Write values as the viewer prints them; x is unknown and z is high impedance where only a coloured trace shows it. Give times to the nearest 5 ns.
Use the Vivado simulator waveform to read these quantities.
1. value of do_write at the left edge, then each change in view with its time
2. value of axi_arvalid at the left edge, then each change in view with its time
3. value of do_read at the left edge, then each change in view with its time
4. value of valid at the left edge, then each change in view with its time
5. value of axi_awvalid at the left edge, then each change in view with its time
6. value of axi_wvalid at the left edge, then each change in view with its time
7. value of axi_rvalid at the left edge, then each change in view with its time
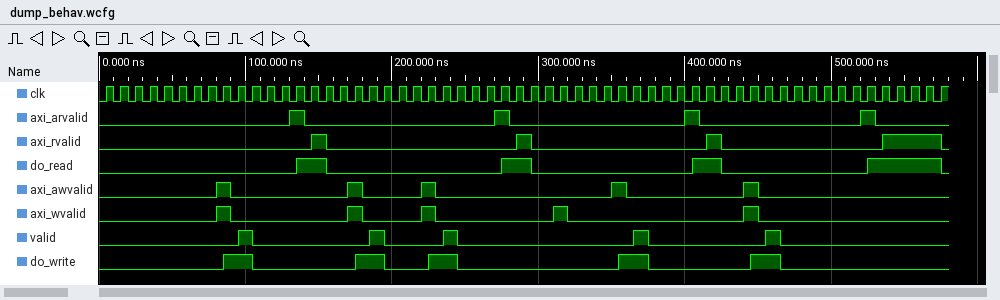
0, 1 at 85 ns, 0 at 105 ns, 1 at 175 ns, 0 at 195 ns, 1 at 225 ns, 0 at 245 ns, 1 at 355 ns, 0 at 375 ns, 1 at 445 ns, 0 at 465 ns
0, 1 at 130 ns, 0 at 140 ns, 1 at 270 ns, 0 at 280 ns, 1 at 400 ns, 0 at 410 ns, 1 at 520 ns, 0 at 530 ns
0, 1 at 135 ns, 0 at 155 ns, 1 at 275 ns, 0 at 295 ns, 1 at 405 ns, 0 at 425 ns, 1 at 525 ns, 0 at 575 ns
0, 1 at 95 ns, 0 at 105 ns, 1 at 185 ns, 0 at 195 ns, 1 at 235 ns, 0 at 245 ns, 1 at 365 ns, 0 at 375 ns, 1 at 455 ns, 0 at 465 ns
0, 1 at 80 ns, 0 at 90 ns, 1 at 170 ns, 0 at 180 ns, 1 at 220 ns, 0 at 230 ns, 1 at 350 ns, 0 at 360 ns, 1 at 440 ns, 0 at 450 ns
0, 1 at 80 ns, 0 at 90 ns, 1 at 170 ns, 0 at 180 ns, 1 at 220 ns, 0 at 230 ns, 1 at 310 ns, 0 at 320 ns, 1 at 440 ns, 0 at 450 ns
0, 1 at 145 ns, 0 at 155 ns, 1 at 285 ns, 0 at 295 ns, 1 at 415 ns, 0 at 425 ns, 1 at 535 ns, 0 at 575 ns
